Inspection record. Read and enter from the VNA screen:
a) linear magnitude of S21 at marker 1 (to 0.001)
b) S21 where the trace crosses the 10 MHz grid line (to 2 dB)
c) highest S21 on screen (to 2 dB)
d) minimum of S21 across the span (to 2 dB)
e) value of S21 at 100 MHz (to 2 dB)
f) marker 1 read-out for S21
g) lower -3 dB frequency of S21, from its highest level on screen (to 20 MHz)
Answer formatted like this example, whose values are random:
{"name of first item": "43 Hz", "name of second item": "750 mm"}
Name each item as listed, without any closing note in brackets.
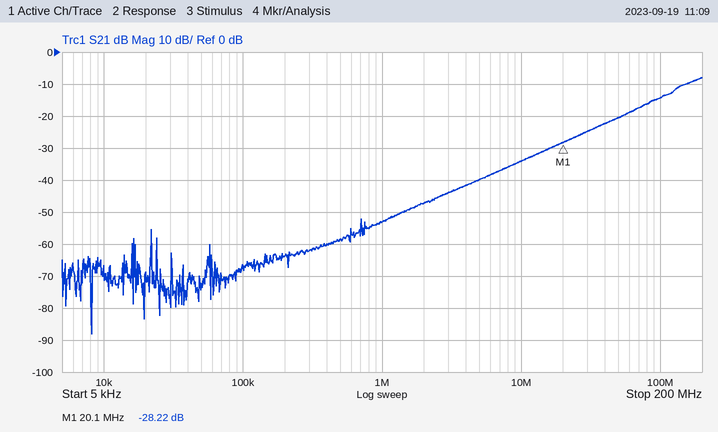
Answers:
{"linear magnitude of S21 at marker 1": "0.039", "S21 where the trace crosses the 10 MHz grid line": "-34 dB", "highest S21 on screen": "-8 dB", "minimum of S21 across the span": "-88 dB", "value of S21 at 100 MHz": "-14 dB", "marker 1 read-out for S21": "-28.22 dB", "lower -3 dB frequency of S21, from its highest level on screen": "140 MHz"}
